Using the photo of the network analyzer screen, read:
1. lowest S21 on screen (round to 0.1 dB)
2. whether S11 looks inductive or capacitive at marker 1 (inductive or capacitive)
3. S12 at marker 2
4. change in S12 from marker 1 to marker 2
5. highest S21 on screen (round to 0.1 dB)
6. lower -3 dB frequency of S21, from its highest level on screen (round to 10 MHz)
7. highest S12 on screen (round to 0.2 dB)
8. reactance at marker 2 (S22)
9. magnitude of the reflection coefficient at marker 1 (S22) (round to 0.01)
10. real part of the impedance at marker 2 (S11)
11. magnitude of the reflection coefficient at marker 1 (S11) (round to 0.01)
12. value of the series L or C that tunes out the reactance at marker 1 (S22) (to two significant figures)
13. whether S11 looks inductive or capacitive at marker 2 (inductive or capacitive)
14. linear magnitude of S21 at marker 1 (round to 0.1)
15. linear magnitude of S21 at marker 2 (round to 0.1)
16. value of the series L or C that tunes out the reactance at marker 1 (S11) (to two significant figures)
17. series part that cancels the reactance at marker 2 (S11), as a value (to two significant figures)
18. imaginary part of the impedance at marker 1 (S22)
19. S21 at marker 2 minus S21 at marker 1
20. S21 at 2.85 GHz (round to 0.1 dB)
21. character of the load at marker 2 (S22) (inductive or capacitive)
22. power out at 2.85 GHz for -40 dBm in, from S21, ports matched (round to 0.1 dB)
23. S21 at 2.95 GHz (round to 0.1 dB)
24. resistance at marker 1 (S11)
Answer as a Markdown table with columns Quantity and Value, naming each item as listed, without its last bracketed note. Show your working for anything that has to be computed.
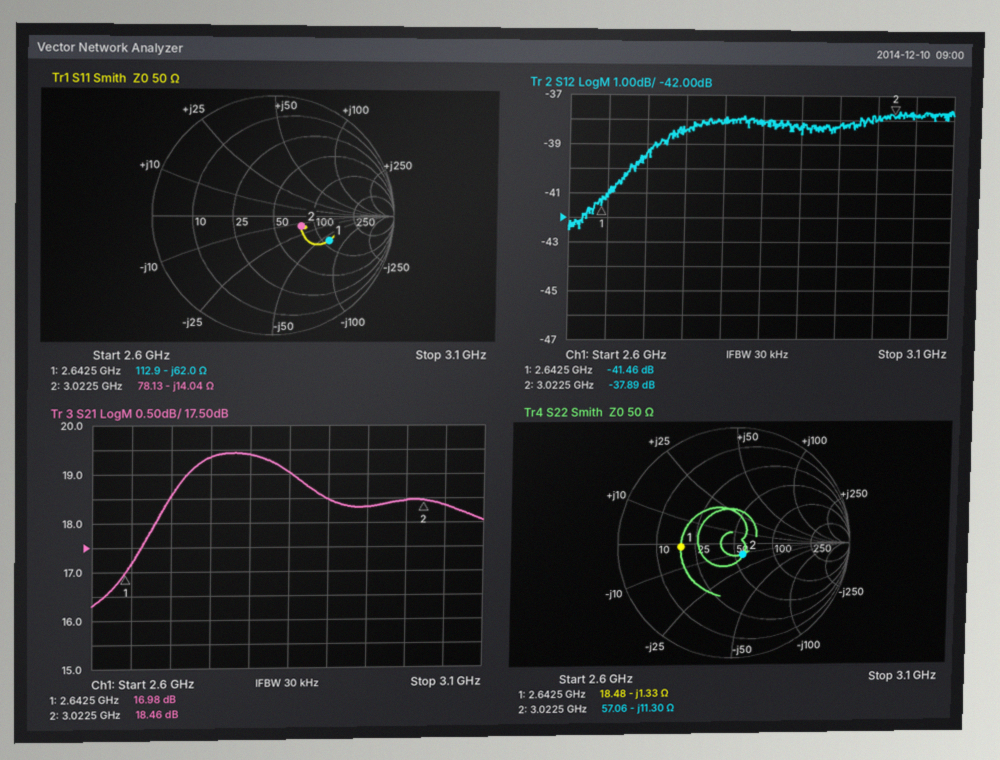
| Quantity | Value |
|---|---|
| lowest S21 on screen | 16.3 dB |
| whether S11 looks inductive or capacitive at marker 1 | capacitive |
| S12 at marker 2 | -37.89 dB |
| change in S12 from marker 1 to marker 2 | -37.89 − (-41.46) = 3.57 dB |
| highest S21 on screen | 19.4 dB |
| lower -3 dB frequency of S21, from its highest level on screen | 2.61 GHz |
| highest S12 on screen | -37.6 dB |
| reactance at marker 2 | -11.30 Ω |
| magnitude of the reflection coefficient at marker 1 (S22) | 0.46 |
| real part of the impedance at marker 2 | 78.13 Ω |
| magnitude of the reflection coefficient at marker 1 (S11) | 0.51 |
| value of the series L or C that tunes out the reactance at marker 1 (S22) | L = 1.33 Ω/(2π × 2.6425 GHz) ≈ 80 pH |
| whether S11 looks inductive or capacitive at marker 2 | capacitive |
| linear magnitude of S21 at marker 1 | 10^(16.98/20) ≈ 7.1 |
| linear magnitude of S21 at marker 2 | 10^(18.46/20) ≈ 8.4 |
| value of the series L or C that tunes out the reactance at marker 1 (S11) | L = 62 Ω/(2π × 2.6425 GHz) ≈ 3.7 nH |
| series part that cancels the reactance at marker 2 (S11), as a value | L = 14.04 Ω/(2π × 3.0225 GHz) ≈ 739 pH, so 740 pH to two significant figures |
| imaginary part of the impedance at marker 1 | -1.33 Ω |
| S21 at marker 2 minus S21 at marker 1 | 18.46 − (16.98) = 1.48 dB |
| S21 at 2.85 GHz | 19.0 dB |
| character of the load at marker 2 (S22) | capacitive |
| power out at 2.85 GHz for -40 dBm in, from S21, ports matched | -40 dBm + (19.0 dB) = -21.0 dBm |
| S21 at 2.95 GHz | 18.3 dB |
| resistance at marker 1 | 112.9 Ω |
